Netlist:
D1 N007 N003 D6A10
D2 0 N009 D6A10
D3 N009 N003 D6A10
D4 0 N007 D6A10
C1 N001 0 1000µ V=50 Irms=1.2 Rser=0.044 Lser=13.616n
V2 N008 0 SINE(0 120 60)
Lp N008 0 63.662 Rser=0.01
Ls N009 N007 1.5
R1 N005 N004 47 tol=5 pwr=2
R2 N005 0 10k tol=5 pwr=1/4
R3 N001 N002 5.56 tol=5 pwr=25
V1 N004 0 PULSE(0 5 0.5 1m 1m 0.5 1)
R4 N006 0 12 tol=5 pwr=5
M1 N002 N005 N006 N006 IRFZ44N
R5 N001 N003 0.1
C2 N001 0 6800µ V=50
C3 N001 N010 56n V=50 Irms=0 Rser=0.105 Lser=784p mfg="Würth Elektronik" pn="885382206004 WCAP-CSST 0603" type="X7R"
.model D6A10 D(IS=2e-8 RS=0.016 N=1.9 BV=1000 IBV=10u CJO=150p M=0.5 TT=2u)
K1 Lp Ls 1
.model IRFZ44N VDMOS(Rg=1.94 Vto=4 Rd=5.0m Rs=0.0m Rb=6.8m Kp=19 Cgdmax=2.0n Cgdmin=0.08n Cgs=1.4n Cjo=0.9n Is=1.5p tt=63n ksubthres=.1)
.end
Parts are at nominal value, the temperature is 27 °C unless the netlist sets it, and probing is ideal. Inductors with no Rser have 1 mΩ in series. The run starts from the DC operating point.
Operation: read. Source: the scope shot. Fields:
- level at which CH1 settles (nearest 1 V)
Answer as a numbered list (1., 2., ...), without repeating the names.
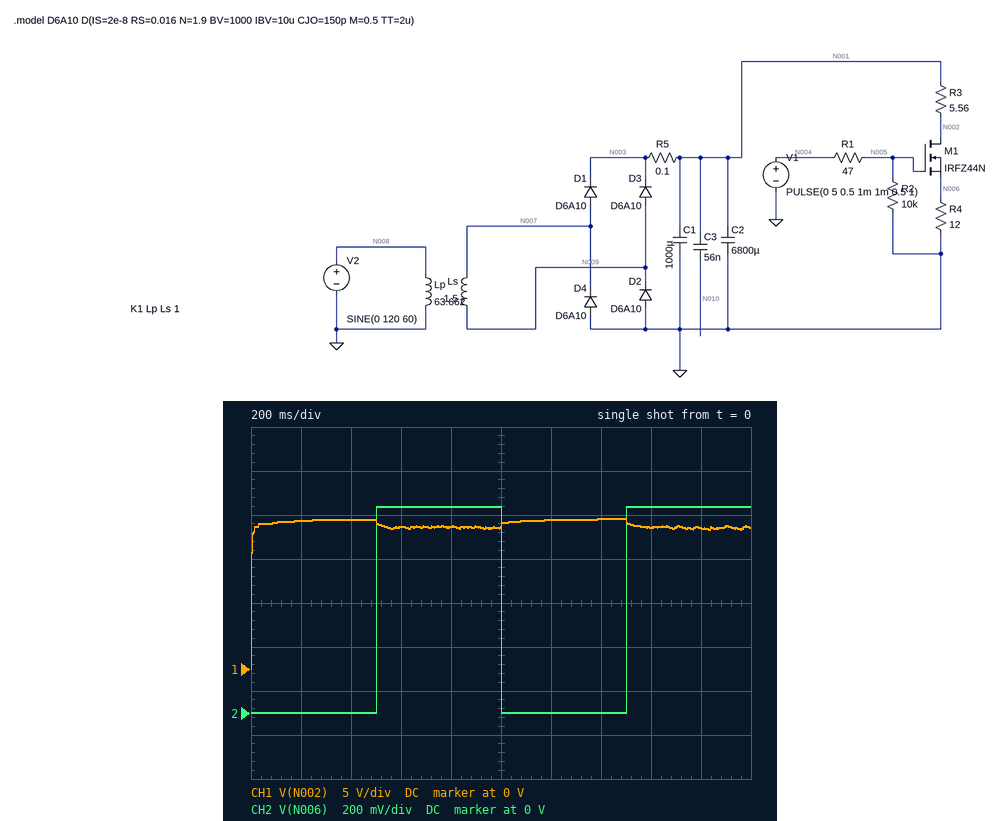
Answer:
1. 16 V
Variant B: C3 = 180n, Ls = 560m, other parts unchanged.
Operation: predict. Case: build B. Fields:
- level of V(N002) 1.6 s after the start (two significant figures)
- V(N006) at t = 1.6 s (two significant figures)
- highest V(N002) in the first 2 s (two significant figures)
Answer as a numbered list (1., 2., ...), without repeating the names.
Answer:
1. 9.0 V
2. 940 mV
3. 9.9 V
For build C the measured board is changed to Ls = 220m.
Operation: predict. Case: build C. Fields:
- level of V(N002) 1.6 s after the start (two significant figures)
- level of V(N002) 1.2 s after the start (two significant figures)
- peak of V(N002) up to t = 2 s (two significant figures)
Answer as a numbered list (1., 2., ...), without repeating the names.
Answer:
1. 4.8 V
2. 5.6 V
3. 5.7 V
